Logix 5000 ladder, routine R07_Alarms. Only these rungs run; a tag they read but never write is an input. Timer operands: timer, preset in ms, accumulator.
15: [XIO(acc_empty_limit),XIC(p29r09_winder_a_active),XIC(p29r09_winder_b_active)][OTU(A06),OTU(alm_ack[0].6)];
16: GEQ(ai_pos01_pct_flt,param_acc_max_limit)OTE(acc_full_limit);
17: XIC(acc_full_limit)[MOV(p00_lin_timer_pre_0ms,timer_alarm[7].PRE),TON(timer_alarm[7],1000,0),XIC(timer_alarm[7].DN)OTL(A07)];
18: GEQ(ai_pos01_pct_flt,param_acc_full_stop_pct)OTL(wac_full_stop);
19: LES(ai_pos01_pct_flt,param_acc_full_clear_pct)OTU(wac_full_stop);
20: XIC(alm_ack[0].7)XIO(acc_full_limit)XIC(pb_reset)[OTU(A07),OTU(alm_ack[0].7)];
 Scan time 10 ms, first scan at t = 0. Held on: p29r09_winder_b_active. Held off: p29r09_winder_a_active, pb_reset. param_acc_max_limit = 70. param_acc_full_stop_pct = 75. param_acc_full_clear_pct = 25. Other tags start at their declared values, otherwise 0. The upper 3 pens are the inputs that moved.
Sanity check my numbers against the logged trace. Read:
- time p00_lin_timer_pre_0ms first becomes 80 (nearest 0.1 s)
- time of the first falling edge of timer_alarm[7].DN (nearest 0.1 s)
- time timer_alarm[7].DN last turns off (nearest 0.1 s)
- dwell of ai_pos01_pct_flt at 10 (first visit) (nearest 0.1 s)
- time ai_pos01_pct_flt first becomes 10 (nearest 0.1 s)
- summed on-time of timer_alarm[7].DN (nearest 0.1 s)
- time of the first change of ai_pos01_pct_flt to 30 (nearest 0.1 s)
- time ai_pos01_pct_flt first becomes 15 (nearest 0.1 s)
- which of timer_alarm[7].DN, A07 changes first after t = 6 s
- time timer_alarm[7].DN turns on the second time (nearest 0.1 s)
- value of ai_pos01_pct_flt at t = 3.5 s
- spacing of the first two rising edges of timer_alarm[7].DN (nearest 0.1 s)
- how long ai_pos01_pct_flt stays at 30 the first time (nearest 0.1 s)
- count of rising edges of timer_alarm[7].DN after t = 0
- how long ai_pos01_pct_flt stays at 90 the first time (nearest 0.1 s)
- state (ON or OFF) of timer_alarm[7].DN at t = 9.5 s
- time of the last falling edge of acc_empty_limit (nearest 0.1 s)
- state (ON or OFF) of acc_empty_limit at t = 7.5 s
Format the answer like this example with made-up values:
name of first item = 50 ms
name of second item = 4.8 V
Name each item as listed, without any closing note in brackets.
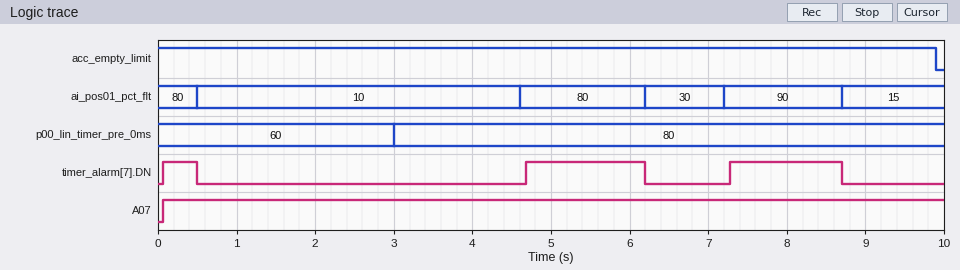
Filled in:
time p00_lin_timer_pre_0ms first becomes 80 = 3.0 s
time of the first falling edge of timer_alarm[7].DN = 0.5 s
time timer_alarm[7].DN last turns off = 8.7 s
dwell of ai_pos01_pct_flt at 10 (first visit) = 4.1 s
time ai_pos01_pct_flt first becomes 10 = 0.5 s
summed on-time of timer_alarm[7].DN = 3.4 s
time of the first change of ai_pos01_pct_flt to 30 = 6.2 s
time ai_pos01_pct_flt first becomes 15 = 8.7 s
which of timer_alarm[7].DN, A07 changes first after t = 6 s = timer_alarm[7].DN
time timer_alarm[7].DN turns on the second time = 4.7 s
value of ai_pos01_pct_flt at t = 3.5 s = 10
spacing of the first two rising edges of timer_alarm[7].DN = 4.6 s
how long ai_pos01_pct_flt stays at 30 the first time = 1.0 s
count of rising edges of timer_alarm[7].DN after t = 0 = 3
how long ai_pos01_pct_flt stays at 90 the first time = 1.5 s
state (ON or OFF) of timer_alarm[7].DN at t = 9.5 s = OFF
time of the last falling edge of acc_empty_limit = 9.9 s
state (ON or OFF) of acc_empty_limit at t = 7.5 s = ON
